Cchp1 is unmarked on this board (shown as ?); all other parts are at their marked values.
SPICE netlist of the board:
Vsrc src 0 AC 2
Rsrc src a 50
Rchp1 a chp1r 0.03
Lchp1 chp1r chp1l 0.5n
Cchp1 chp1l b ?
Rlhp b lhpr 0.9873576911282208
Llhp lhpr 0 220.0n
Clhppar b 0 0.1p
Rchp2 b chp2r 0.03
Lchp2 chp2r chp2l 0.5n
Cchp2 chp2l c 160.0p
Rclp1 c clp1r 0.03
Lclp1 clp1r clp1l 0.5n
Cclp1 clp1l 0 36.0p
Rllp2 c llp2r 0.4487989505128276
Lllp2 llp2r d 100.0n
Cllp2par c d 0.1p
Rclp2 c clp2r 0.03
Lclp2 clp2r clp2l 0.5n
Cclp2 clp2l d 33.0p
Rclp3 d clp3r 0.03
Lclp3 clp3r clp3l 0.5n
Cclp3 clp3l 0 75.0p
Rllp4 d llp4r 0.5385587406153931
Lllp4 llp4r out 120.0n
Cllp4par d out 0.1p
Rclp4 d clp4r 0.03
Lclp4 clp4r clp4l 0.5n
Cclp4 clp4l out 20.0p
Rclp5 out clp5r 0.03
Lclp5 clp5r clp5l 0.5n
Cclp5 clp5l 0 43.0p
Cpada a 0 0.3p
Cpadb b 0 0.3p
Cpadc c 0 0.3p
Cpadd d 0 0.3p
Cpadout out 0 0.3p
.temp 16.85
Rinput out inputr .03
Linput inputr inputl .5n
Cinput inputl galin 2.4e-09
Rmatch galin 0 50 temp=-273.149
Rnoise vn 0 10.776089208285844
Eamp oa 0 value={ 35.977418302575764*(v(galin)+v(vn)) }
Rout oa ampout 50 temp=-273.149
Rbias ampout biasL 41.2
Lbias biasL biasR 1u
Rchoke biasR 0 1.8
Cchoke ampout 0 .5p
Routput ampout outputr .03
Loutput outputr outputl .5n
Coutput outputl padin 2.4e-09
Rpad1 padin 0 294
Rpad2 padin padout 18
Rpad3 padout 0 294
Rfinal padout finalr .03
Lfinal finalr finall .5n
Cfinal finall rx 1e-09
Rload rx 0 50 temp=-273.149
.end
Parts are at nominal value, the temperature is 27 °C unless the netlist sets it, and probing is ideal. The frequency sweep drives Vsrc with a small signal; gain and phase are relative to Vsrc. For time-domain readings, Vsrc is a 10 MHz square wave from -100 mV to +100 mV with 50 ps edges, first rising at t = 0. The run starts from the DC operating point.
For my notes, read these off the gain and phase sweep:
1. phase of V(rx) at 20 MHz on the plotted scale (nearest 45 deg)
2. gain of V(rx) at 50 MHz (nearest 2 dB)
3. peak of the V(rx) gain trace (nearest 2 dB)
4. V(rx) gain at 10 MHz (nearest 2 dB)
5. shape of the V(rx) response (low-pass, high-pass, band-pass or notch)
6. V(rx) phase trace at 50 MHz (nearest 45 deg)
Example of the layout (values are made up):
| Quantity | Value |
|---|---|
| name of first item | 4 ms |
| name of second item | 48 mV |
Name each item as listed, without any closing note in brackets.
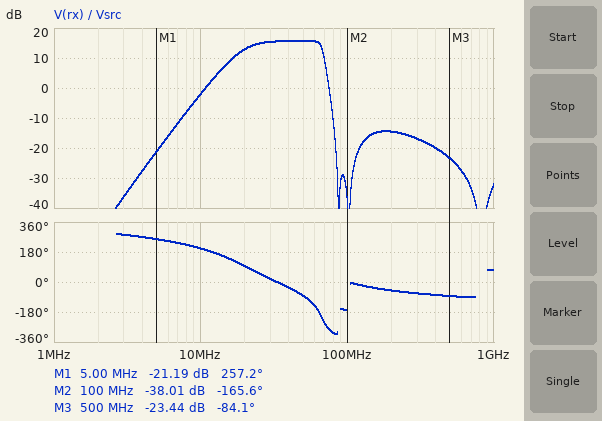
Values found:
| Quantity | Value |
|---|---|
| phase of V(rx) at 20 MHz on the plotted scale | 90 deg |
| gain of V(rx) at 50 MHz | 16 dB |
| peak of the V(rx) gain trace | 16 dB |
| V(rx) gain at 10 MHz | -2 dB |
| shape of the V(rx) response | band-pass |
| V(rx) phase trace at 50 MHz | -90 deg |
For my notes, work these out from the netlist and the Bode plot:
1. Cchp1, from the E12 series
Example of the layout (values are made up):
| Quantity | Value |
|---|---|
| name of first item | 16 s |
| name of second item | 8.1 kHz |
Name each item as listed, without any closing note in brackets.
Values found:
| Quantity | Value |
|---|---|
| Cchp1, from the E12 series | 220 pF |
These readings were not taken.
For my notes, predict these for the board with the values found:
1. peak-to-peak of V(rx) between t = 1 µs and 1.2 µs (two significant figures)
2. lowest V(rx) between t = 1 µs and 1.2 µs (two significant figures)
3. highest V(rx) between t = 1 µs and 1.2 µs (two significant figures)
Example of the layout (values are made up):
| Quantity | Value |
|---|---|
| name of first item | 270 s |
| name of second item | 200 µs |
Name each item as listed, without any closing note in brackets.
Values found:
| Quantity | Value |
|---|---|
| peak-to-peak of V(rx) between t = 1 µs and 1.2 µs | 1.0 V |
| lowest V(rx) between t = 1 µs and 1.2 µs | -520 mV |
| highest V(rx) between t = 1 µs and 1.2 µs | 520 mV |
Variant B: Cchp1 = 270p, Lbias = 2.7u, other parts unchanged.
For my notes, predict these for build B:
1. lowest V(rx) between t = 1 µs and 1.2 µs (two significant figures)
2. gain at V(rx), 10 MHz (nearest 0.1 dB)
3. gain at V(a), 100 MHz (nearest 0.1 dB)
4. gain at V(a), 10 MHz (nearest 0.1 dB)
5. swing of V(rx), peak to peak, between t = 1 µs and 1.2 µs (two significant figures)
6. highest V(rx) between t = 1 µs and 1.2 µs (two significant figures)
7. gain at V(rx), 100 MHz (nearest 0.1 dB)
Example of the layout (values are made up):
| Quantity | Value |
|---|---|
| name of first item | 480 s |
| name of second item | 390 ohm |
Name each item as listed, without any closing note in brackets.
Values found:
| Quantity | Value |
|---|---|
| lowest V(rx) between t = 1 µs and 1.2 µs | -540 mV |
| gain at V(rx), 10 MHz | 0.4 dB |
| gain at V(a), 100 MHz | -1.7 dB |
| gain at V(a), 10 MHz | -3.8 dB |
| swing of V(rx), peak to peak, between t = 1 µs and 1.2 µs | 1.1 V |
| highest V(rx) between t = 1 µs and 1.2 µs | 540 mV |
| gain at V(rx), 100 MHz | -37.9 dB |
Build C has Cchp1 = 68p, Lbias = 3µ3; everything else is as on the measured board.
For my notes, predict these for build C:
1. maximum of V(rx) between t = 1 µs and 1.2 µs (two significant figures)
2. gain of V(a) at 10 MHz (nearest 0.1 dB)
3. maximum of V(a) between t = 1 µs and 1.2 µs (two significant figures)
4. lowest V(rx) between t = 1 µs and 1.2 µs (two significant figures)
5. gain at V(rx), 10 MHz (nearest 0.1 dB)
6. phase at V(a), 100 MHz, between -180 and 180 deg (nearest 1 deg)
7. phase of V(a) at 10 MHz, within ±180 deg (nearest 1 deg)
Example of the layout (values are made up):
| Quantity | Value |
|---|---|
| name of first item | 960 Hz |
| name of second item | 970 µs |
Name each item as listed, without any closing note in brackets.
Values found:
| Quantity | Value |
|---|---|
| maximum of V(rx) between t = 1 µs and 1.2 µs | 470 mV |
| gain of V(a) at 10 MHz | -0.2 dB |
| maximum of V(a) between t = 1 µs and 1.2 µs | 110 mV |
| lowest V(rx) between t = 1 µs and 1.2 µs | -470 mV |
| gain at V(rx), 10 MHz | -9.9 dB |
| phase at V(a), 100 MHz, between -180 and 180 deg | -29 deg |
| phase of V(a) at 10 MHz, within ±180 deg | -13 deg |
